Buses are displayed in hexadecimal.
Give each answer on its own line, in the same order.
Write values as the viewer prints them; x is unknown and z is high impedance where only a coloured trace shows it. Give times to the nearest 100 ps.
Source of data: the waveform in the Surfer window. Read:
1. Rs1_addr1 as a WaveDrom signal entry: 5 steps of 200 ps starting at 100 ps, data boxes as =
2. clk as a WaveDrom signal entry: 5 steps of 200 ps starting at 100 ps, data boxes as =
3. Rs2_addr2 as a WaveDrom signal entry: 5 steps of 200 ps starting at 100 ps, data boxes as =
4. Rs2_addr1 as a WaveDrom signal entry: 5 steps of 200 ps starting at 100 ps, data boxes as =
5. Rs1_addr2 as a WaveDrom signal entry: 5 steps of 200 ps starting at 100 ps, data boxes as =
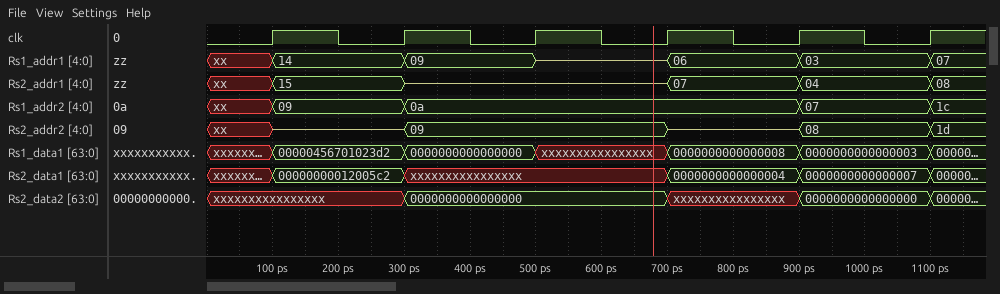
{name: 'Rs1_addr1', wave: '==z==', data: '14 09 06 03'}
{name: 'clk', wave: 'p....'}
{name: 'Rs2_addr2', wave: 'z=.z=', data: '09 08'}
{name: 'Rs2_addr1', wave: '=z.==', data: '15 07 04'}
{name: 'Rs1_addr2', wave: '==..=', data: '09 0a 07'}
